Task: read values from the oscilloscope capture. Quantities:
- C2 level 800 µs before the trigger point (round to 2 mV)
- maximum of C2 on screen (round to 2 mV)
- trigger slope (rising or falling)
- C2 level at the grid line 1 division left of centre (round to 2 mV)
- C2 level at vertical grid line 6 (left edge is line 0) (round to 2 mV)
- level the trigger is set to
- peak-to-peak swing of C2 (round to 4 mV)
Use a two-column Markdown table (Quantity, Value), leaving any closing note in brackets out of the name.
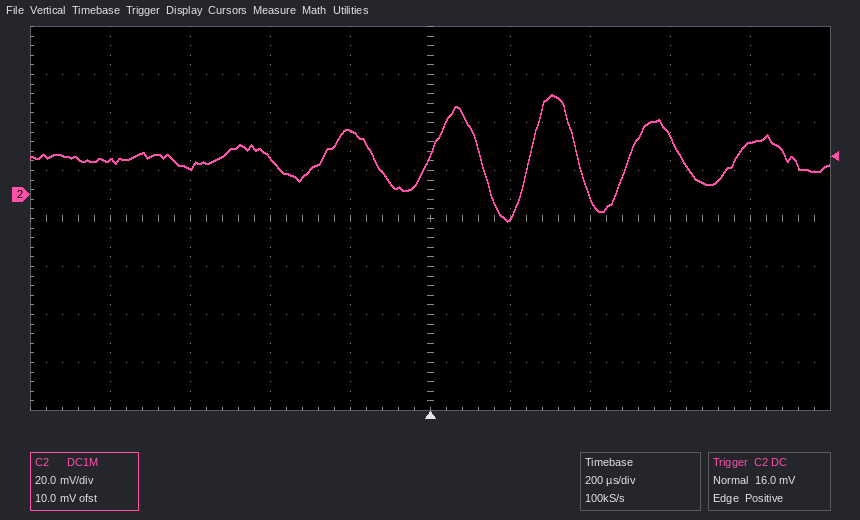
| Quantity | Value |
|---|---|
| C2 level 800 µs before the trigger point | 14 mV |
| maximum of C2 on screen | 42 mV |
| trigger slope | rising |
| C2 level at the grid line 1 division left of centre | 26 mV |
| C2 level at vertical grid line 6 (left edge is line 0) | -10 mV |
| level the trigger is set to | 16.0 mV |
| peak-to-peak swing of C2 | 52 mV |
